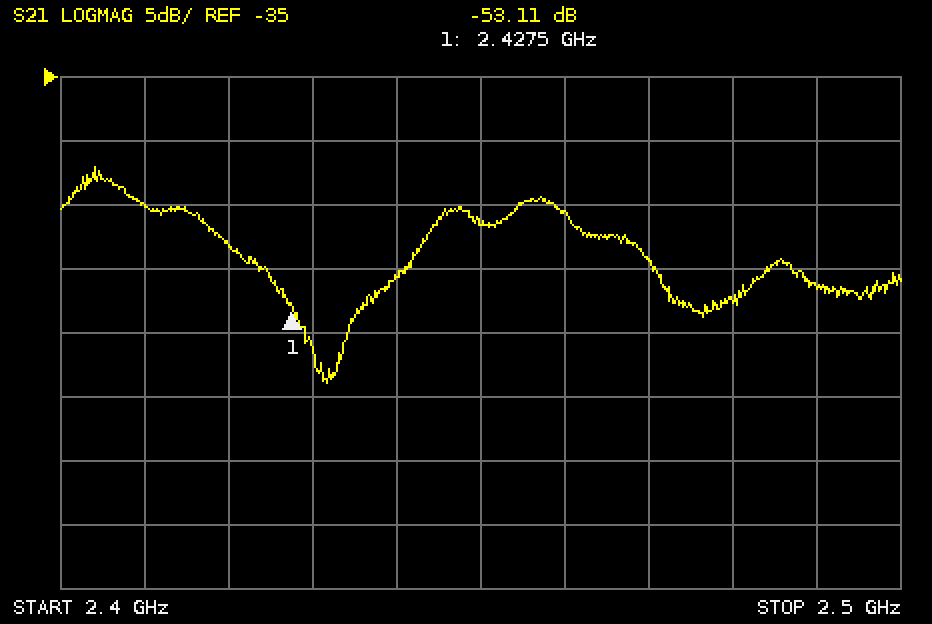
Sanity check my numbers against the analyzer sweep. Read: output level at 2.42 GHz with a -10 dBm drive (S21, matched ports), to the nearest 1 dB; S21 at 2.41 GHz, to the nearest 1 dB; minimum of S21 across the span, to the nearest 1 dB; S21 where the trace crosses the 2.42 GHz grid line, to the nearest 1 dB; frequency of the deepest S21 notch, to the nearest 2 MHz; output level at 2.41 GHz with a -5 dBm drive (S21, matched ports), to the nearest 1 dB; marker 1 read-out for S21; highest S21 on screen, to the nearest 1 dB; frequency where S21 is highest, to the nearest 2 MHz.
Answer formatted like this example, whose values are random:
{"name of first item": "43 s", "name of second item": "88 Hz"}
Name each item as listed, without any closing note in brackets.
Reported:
{"output level at 2.42 GHz with a -10 dBm drive (S21, matched ports), to the nearest 1 dB": "-58 dBm", "S21 at 2.41 GHz, to the nearest 1 dB": "-45 dB", "minimum of S21 across the span, to the nearest 1 dB": "-59 dB", "S21 where the trace crosses the 2.42 GHz grid line, to the nearest 1 dB": "-48 dB", "frequency of the deepest S21 notch, to the nearest 2 MHz": "2.432 GHz", "output level at 2.41 GHz with a -5 dBm drive (S21, matched ports), to the nearest 1 dB": "-50 dBm", "marker 1 read-out for S21": "-53.11 dB", "highest S21 on screen, to the nearest 1 dB": "-42 dB", "frequency where S21 is highest, to the nearest 2 MHz": "2.404 GHz"}
